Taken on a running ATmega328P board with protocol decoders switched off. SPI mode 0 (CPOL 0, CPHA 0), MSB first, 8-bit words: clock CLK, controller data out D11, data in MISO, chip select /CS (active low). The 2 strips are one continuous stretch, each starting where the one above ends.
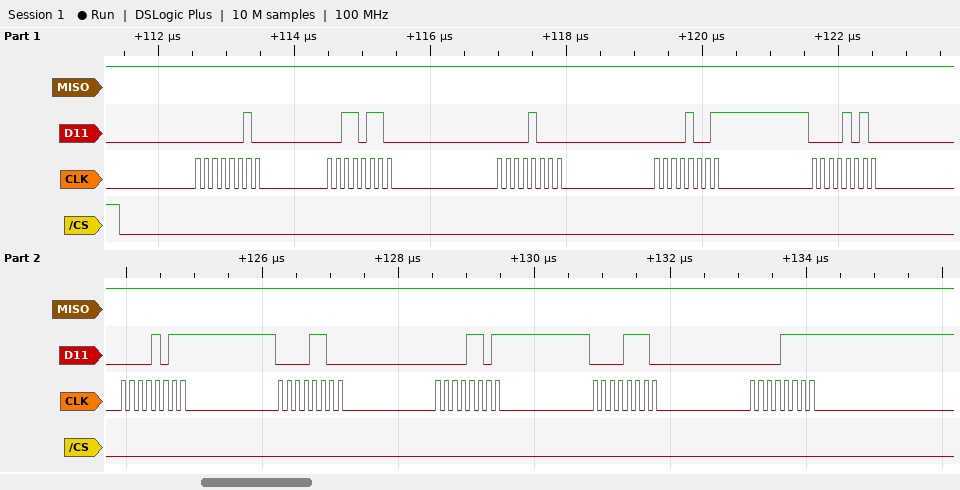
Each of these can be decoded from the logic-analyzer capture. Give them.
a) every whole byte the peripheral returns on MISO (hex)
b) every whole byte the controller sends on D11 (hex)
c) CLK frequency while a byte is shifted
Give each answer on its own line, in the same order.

FF FF FF FF FF FF FF FF FF FF
02 36 08 09 0A 0B 0C 0D 0E 0F
8 MHz
